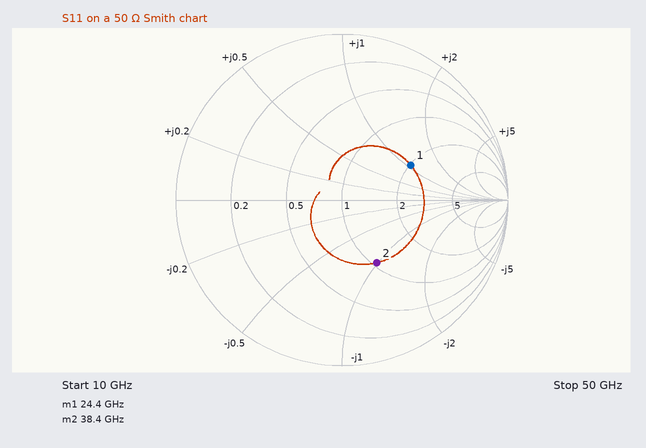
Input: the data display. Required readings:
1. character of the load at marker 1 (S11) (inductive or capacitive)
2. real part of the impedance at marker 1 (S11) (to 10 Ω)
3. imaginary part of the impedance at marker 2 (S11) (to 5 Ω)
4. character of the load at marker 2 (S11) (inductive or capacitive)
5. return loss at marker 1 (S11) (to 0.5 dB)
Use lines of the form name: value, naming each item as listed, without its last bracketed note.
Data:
character of the load at marker 1 (S11): inductive
real part of the impedance at marker 1 (S11): 100 Ω
imaginary part of the impedance at marker 2 (S11): -50 Ω
character of the load at marker 2 (S11): capacitive
return loss at marker 1 (S11): 6.5 dB
